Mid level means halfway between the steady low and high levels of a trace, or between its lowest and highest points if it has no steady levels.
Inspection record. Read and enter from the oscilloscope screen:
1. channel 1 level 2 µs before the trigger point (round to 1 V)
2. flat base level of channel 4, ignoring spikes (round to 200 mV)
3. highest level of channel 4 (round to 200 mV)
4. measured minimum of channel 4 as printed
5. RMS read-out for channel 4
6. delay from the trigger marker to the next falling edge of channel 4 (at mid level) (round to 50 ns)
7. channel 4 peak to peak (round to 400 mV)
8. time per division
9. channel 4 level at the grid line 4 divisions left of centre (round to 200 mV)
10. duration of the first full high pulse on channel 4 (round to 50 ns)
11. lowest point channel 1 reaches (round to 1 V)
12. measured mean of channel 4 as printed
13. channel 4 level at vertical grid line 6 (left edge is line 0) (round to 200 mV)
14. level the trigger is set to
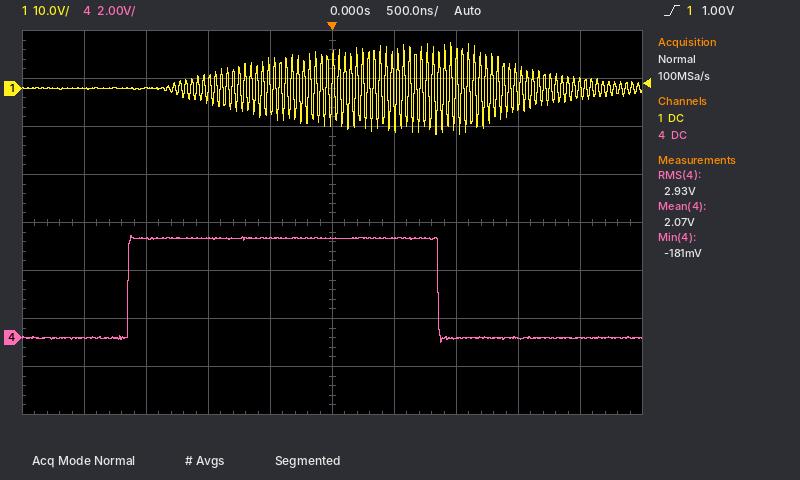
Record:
0 V
0.0 V
4.2 V
-181 mV
2.93 V
850 ns
4.4 V
500 ns
0.0 V
2.50 µs
-10 V
2.07 V
4.2 V
1.00 V
